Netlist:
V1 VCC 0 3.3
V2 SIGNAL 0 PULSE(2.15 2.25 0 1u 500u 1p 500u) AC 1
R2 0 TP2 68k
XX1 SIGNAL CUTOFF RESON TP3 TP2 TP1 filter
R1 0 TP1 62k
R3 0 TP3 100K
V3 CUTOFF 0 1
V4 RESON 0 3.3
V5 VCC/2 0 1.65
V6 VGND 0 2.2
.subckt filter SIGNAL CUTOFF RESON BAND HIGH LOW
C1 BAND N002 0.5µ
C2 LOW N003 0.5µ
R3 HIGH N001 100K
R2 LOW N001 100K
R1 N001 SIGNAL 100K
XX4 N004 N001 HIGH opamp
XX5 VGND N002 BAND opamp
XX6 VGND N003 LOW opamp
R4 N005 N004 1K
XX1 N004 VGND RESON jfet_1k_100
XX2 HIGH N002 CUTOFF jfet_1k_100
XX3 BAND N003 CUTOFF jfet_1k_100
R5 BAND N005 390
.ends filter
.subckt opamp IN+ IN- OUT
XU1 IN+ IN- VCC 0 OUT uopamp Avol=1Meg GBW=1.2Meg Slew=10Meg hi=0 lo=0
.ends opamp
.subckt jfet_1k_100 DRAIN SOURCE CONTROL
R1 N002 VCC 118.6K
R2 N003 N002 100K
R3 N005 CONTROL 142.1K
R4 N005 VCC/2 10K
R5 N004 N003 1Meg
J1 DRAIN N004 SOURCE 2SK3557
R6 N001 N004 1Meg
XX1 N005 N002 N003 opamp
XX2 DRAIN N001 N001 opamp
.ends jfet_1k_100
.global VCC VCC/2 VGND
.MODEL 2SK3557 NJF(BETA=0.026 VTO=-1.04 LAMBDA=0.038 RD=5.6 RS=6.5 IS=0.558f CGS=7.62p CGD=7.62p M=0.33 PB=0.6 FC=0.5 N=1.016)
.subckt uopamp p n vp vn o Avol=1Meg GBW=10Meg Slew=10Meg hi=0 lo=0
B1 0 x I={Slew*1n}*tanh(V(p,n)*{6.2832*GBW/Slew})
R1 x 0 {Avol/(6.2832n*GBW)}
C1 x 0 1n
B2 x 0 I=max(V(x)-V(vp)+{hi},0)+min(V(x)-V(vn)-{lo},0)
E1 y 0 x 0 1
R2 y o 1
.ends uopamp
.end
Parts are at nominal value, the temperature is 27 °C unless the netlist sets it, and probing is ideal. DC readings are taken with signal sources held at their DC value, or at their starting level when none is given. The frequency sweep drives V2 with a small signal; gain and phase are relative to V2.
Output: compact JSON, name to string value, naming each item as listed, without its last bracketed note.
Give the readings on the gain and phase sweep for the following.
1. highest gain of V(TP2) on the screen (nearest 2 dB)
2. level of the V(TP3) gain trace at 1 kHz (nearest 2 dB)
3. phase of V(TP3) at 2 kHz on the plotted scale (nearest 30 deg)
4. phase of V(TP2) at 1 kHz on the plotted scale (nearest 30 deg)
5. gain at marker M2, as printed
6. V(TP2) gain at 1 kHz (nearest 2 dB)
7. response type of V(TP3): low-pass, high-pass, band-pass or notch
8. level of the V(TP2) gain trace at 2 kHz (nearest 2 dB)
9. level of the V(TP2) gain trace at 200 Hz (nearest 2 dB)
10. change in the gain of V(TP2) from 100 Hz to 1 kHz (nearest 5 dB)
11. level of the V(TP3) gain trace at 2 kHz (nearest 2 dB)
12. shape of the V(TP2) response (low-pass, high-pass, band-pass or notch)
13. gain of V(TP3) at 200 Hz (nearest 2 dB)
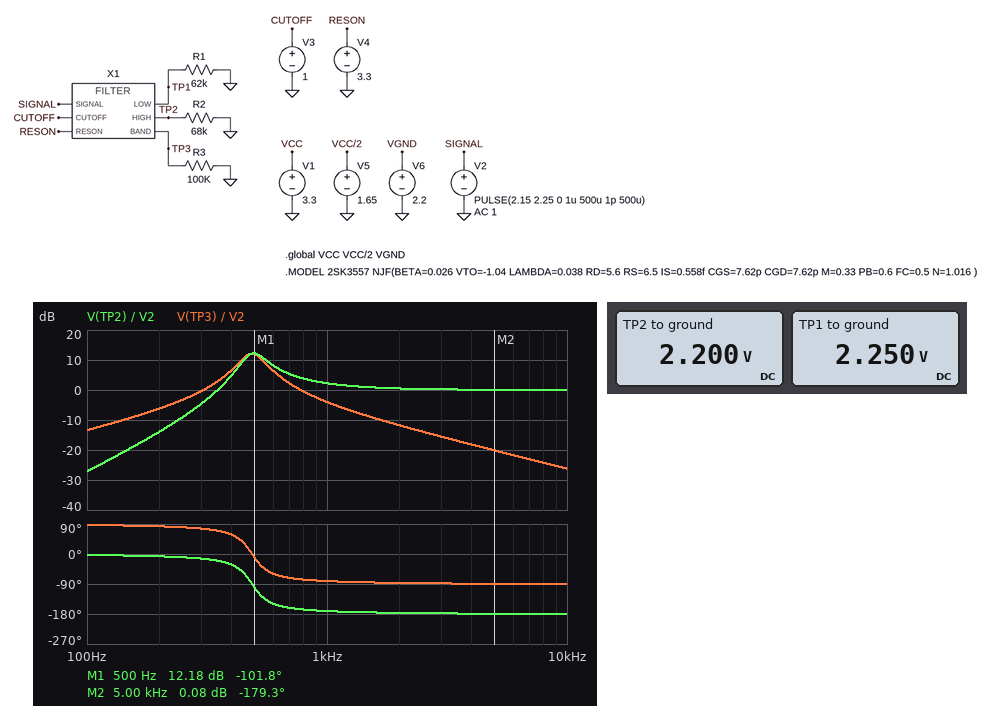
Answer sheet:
{"highest gain of V(TP2) on the screen": "12 dB", "level of the V(TP3) gain trace at 1 kHz": "-4 dB", "phase of V(TP3) at 2 kHz on the plotted scale": "-90 deg", "phase of V(TP2) at 1 kHz on the plotted scale": "-180 deg", "gain at marker M2, as printed": "0.08 dB", "V(TP2) gain at 1 kHz": "2 dB", "response type of V(TP3): low-pass, high-pass, band-pass or notch": "band-pass", "level of the V(TP2) gain trace at 2 kHz": "0 dB", "level of the V(TP2) gain trace at 200 Hz": "-14 dB", "change in the gain of V(TP2) from 100 Hz to 1 kHz": "30 dB", "level of the V(TP3) gain trace at 2 kHz": "-12 dB", "shape of the V(TP2) response": "high-pass", "gain of V(TP3) at 200 Hz": "-6 dB"}
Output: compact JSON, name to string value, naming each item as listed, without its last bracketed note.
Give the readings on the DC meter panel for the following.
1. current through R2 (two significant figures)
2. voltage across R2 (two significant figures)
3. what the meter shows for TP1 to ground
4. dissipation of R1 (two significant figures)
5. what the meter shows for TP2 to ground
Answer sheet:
{"current through R2": "32 µA", "voltage across R2": "2.2 V", "what the meter shows for TP1 to ground": "2.250 V", "dissipation of R1": "82 µW", "what the meter shows for TP2 to ground": "2.200 V"}
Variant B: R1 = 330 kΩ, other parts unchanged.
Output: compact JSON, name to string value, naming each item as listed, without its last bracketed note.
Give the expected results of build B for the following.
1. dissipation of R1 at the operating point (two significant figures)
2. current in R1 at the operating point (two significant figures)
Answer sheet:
{"dissipation of R1 at the operating point": "15 µW", "current in R1 at the operating point": "6.8 µA"}
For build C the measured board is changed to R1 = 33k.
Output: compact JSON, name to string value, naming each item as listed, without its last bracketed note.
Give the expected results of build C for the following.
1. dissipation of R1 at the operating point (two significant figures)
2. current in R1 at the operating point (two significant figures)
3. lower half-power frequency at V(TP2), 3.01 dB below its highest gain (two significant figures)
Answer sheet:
{"dissipation of R1 at the operating point": "150 µW", "current in R1 at the operating point": "68 µA", "lower half-power frequency at V(TP2), 3.01 dB below its highest gain": "440 Hz"}
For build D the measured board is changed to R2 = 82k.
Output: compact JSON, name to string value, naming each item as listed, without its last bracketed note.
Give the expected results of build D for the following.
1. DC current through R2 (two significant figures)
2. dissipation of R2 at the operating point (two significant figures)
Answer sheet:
{"DC current through R2": "27 µA", "dissipation of R2 at the operating point": "59 µW"}
